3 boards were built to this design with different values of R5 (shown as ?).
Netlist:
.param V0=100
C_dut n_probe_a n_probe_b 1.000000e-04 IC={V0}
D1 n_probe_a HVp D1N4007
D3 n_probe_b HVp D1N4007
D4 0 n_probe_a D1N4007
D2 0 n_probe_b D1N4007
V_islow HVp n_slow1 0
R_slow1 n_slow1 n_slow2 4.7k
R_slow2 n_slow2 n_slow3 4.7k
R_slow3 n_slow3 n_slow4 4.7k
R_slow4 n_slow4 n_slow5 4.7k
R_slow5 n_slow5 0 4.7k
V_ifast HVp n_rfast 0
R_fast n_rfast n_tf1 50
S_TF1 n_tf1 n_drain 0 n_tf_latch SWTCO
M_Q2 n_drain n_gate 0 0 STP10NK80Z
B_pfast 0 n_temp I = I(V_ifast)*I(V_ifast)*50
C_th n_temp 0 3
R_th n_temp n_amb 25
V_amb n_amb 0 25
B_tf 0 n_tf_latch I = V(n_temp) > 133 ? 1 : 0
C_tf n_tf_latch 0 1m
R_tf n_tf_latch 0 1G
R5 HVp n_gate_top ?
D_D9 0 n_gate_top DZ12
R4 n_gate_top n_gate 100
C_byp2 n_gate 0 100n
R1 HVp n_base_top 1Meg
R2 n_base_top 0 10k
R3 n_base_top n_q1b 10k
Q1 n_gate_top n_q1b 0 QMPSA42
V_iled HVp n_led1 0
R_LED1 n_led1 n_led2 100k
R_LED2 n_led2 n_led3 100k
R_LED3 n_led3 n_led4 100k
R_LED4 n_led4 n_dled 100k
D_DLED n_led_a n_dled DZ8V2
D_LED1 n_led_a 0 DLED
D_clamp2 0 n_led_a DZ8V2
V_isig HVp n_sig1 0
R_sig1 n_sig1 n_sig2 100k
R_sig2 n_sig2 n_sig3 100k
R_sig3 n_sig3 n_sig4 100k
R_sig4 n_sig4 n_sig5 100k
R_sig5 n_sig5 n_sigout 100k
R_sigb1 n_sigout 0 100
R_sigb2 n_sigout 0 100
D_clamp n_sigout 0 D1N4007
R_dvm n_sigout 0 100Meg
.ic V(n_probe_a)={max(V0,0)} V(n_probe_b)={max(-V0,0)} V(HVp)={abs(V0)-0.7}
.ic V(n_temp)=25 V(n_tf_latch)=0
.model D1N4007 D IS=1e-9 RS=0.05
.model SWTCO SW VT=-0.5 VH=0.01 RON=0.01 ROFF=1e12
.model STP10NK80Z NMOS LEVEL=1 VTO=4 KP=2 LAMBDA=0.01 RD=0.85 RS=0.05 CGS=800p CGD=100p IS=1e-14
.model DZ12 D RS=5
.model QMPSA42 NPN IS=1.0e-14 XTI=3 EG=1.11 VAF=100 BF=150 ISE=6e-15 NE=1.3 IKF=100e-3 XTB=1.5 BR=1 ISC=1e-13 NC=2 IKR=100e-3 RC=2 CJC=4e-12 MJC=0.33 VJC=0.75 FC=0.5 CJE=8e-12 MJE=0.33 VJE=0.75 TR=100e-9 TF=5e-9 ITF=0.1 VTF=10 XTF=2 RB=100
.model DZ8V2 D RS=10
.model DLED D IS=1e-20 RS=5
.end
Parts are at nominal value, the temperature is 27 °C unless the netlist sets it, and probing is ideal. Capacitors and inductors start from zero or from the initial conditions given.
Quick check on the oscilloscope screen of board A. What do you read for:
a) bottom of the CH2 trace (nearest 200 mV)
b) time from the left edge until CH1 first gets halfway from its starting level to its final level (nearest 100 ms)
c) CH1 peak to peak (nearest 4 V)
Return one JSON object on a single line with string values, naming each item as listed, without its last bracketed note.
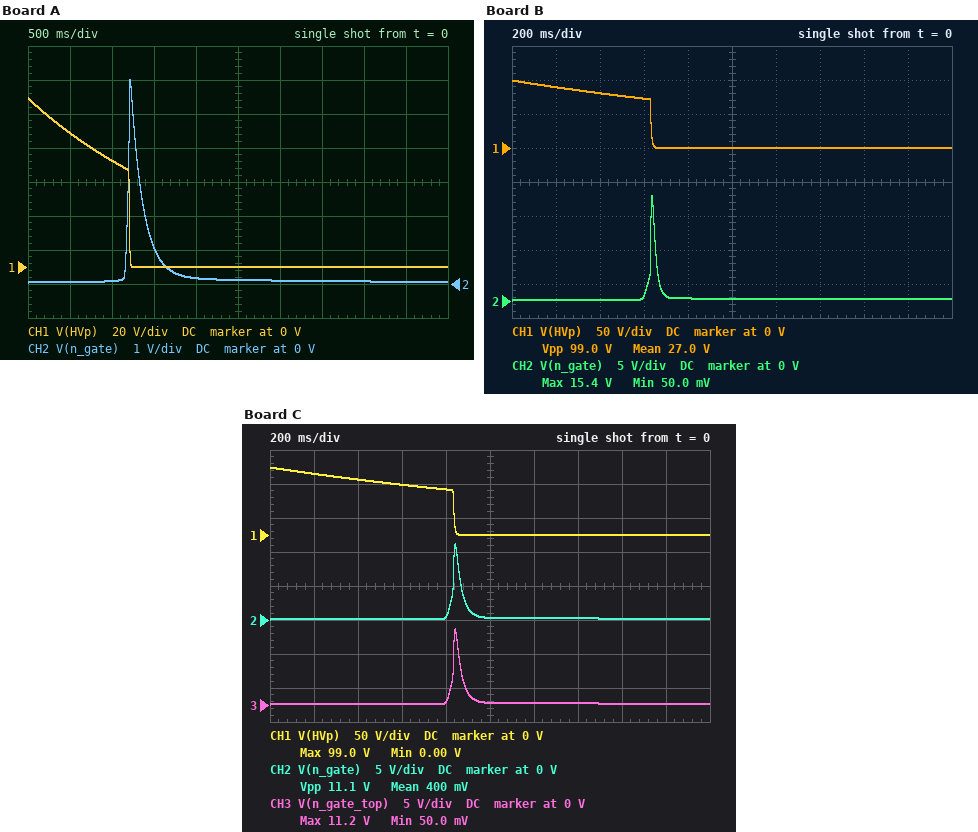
{"bottom of the CH2 trace": "0 V", "time from the left edge until CH1 first gets halfway from its starting level to its final level": "1.2 s", "CH1 peak to peak": "100 V"}
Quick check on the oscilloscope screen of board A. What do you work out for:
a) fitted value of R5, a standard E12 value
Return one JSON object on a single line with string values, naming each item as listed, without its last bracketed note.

{"fitted value of R5, a standard E12 value": "1.5 MΩ"}
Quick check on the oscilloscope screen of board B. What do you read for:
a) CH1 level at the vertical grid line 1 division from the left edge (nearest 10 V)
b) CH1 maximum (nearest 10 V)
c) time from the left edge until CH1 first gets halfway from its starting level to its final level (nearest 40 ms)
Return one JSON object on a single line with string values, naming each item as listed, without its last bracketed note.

{"CH1 level at the vertical grid line 1 division from the left edge": "90 V", "CH1 maximum": "100 V", "time from the left edge until CH1 first gets halfway from its starting level to its final level": "640 ms"}
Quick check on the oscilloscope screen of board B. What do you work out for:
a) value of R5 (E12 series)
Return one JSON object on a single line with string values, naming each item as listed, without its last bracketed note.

{"value of R5": "150 kΩ"}
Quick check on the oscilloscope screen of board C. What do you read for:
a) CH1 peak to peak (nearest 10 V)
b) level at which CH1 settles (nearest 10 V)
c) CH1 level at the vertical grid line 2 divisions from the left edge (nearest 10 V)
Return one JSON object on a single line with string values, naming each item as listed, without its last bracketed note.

{"CH1 peak to peak": "100 V", "level at which CH1 settles": "0 V", "CH1 level at the vertical grid line 2 divisions from the left edge": "80 V"}
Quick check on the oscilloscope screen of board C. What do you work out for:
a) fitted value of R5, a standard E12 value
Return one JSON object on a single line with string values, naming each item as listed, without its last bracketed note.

{"fitted value of R5, a standard E12 value": "270 kΩ"}
